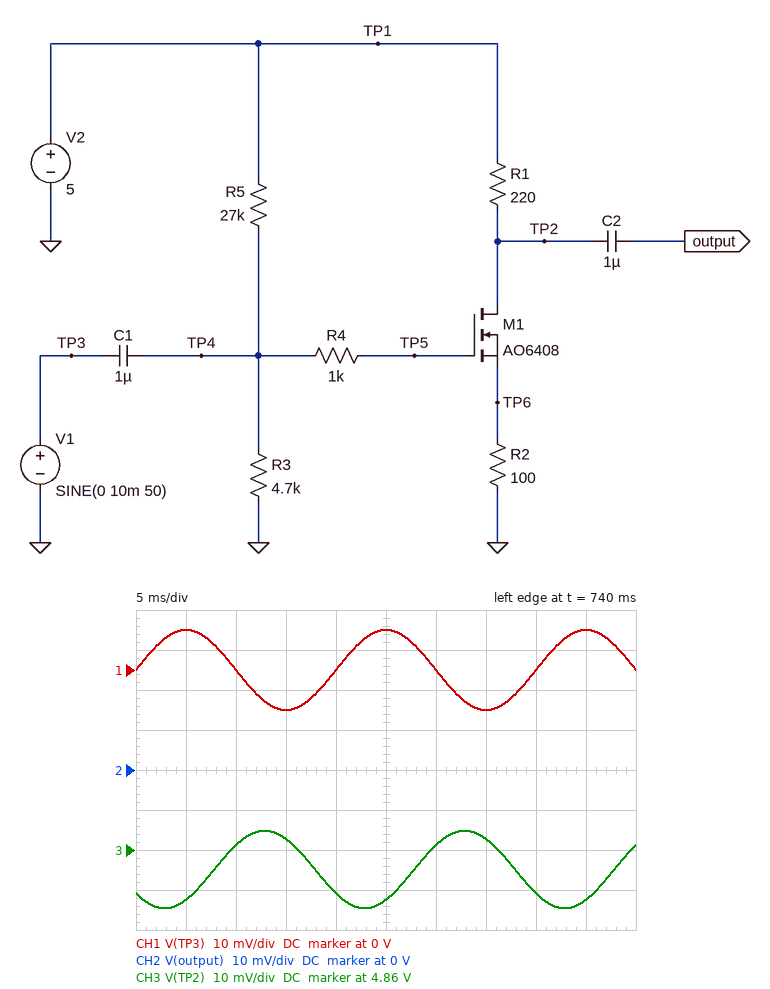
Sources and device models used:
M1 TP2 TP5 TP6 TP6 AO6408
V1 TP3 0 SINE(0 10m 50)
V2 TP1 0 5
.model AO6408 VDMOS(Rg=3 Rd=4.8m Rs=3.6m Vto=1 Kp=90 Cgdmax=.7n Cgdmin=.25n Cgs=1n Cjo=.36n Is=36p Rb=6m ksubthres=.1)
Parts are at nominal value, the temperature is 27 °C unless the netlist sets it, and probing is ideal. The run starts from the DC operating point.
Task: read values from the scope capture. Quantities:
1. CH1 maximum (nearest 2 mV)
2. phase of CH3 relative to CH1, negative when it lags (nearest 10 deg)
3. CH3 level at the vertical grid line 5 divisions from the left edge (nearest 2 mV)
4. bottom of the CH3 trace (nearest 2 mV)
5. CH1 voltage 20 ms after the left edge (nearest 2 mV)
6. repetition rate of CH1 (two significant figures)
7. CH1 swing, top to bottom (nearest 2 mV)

10 mV
-140 deg
4.848 V
4.846 V
0 V
50 Hz
20 mV
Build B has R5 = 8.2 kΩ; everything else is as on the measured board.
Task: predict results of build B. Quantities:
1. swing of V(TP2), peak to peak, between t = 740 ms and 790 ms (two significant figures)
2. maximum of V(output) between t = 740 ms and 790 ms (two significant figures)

29 mV
2.8 V
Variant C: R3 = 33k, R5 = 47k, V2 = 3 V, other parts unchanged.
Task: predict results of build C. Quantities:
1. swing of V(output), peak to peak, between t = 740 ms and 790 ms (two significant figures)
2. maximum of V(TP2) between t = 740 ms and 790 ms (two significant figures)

39 mV
2.0 V
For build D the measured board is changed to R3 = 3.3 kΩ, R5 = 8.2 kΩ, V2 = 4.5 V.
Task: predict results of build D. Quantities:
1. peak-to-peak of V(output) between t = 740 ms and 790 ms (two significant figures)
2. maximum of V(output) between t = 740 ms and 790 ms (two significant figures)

24 mV
3.4 V
